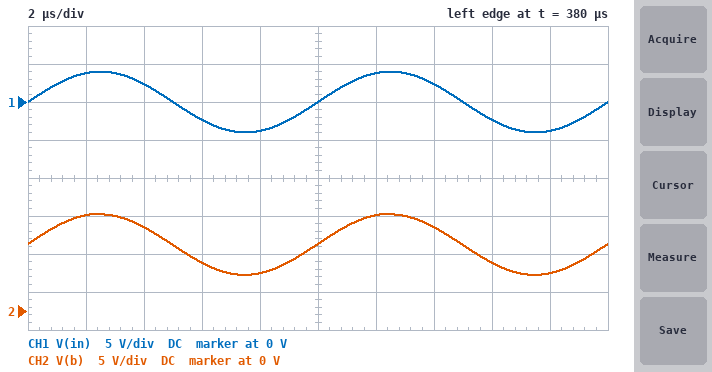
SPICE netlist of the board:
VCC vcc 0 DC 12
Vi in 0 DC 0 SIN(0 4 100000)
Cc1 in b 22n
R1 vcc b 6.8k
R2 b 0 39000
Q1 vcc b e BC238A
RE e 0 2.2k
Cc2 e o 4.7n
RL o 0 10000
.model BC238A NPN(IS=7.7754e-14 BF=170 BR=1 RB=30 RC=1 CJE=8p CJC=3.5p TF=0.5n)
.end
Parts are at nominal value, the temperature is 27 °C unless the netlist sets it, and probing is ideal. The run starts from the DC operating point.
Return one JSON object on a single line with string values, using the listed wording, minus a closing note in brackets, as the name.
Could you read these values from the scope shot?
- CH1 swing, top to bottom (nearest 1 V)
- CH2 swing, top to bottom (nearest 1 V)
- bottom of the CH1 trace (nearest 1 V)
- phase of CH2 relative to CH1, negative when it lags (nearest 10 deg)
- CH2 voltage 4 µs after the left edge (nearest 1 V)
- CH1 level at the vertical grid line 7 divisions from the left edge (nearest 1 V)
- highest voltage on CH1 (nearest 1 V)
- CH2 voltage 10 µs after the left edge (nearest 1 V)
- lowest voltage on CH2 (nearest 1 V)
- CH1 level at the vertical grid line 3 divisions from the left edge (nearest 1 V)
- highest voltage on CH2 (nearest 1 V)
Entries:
{"CH1 swing, top to bottom": "8 V", "CH2 swing, top to bottom": "8 V", "bottom of the CH1 trace": "-4 V", "phase of CH2 relative to CH1, negative when it lags": "0 deg", "CH2 voltage 4 µs after the left edge": "11 V", "CH1 level at the vertical grid line 7 divisions from the left edge": "2 V", "highest voltage on CH1": "4 V", "CH2 voltage 10 µs after the left edge": "9 V", "lowest voltage on CH2": "5 V", "CH1 level at the vertical grid line 3 divisions from the left edge": "-2 V", "highest voltage on CH2": "13 V"}
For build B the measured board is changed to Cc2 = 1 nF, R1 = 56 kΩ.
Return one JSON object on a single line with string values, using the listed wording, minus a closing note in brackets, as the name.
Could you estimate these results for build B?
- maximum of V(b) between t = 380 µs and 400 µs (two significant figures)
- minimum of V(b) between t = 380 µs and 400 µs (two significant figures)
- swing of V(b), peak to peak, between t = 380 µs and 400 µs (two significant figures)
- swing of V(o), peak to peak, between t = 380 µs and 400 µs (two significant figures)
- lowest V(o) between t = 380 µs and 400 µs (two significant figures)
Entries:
{"maximum of V(b) between t = 380 µs and 400 µs": "8.7 V", "minimum of V(b) between t = 380 µs and 400 µs": "670 mV", "swing of V(b), peak to peak, between t = 380 µs and 400 µs": "8.0 V", "swing of V(o), peak to peak, between t = 380 µs and 400 µs": "7.4 V", "lowest V(o) between t = 380 µs and 400 µs": "-3.6 V"}
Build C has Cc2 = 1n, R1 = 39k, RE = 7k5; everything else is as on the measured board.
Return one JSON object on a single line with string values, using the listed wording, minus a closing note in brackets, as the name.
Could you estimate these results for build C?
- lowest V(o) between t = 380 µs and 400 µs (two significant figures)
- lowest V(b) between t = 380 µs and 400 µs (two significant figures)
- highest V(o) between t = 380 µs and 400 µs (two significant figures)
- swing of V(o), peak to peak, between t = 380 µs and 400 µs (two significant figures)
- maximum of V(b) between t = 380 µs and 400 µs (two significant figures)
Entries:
{"lowest V(o) between t = 380 µs and 400 µs": "-3.3 V", "lowest V(b) between t = 380 µs and 400 µs": "1.9 V", "highest V(o) between t = 380 µs and 400 µs": "3.8 V", "swing of V(o), peak to peak, between t = 380 µs and 400 µs": "7.1 V", "maximum of V(b) between t = 380 µs and 400 µs": "9.9 V"}
